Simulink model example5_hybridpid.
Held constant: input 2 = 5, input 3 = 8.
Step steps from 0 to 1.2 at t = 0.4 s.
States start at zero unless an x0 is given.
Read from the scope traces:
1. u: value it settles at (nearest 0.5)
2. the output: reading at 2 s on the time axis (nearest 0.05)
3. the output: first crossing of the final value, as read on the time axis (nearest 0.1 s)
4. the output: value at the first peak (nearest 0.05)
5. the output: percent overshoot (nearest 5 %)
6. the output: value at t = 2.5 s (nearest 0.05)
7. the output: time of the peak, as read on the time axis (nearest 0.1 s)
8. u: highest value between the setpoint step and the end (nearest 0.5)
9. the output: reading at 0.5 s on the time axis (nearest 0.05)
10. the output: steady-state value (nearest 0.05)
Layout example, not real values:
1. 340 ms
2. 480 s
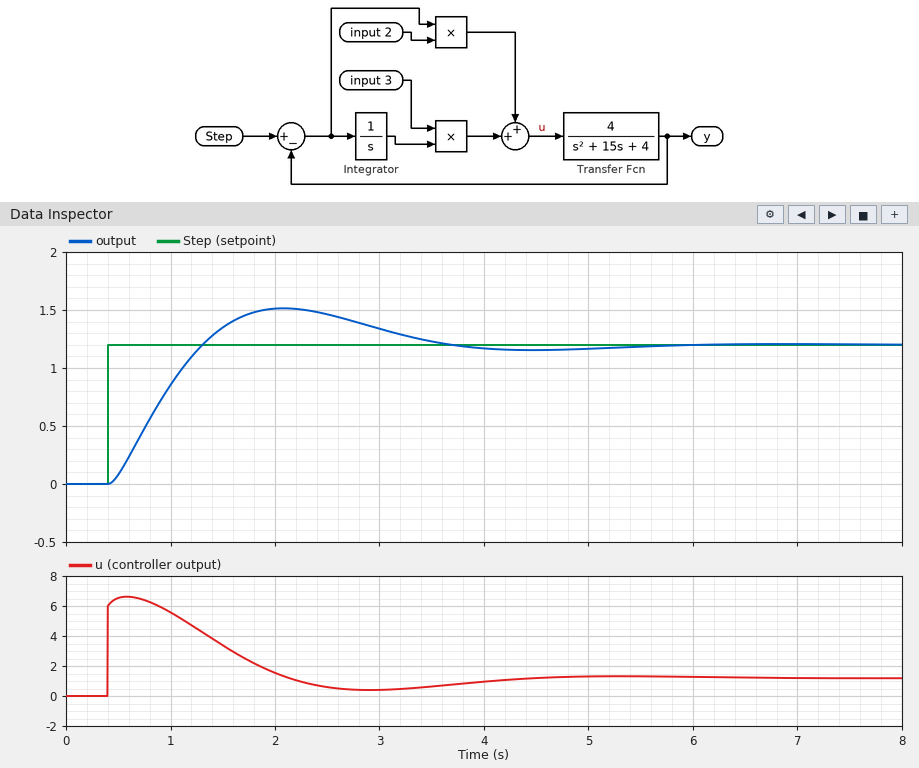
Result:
1. 1.0
2. 1.50
3. 1.3 s
4. 1.50
5. 25 %
6. 1.45
7. 2.1 s
8. 6.5
9. 0.10
10. 1.20
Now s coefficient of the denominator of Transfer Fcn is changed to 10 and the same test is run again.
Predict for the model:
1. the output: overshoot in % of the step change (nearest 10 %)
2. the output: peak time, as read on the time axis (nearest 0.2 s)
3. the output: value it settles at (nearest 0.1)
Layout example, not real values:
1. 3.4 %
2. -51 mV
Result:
1. 20 %
2. 1.6 s
3. 1.2
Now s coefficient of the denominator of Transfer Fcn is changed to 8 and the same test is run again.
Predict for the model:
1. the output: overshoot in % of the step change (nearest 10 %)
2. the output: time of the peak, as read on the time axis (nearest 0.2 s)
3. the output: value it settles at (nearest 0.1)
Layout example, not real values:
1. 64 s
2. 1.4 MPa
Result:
1. 20 %
2. 1.4 s
3. 1.2
